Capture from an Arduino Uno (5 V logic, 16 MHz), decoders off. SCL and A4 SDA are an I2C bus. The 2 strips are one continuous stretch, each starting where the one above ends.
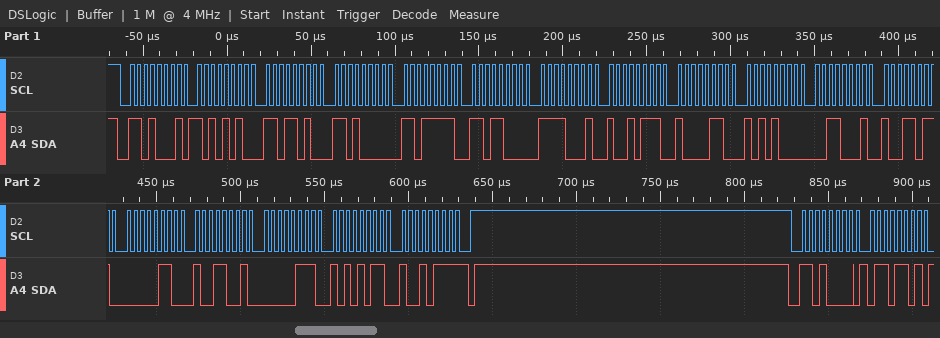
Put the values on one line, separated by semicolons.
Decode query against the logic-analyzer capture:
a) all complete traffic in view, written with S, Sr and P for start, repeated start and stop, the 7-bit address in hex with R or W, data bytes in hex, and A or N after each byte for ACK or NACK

S 68R A AA A DA A D0 A DF A D8 A F1 A 97 A 86 A A8 A 31 A 9B A 06 A 99 A 07 A AB A 97 N P S 68W A 6D A
